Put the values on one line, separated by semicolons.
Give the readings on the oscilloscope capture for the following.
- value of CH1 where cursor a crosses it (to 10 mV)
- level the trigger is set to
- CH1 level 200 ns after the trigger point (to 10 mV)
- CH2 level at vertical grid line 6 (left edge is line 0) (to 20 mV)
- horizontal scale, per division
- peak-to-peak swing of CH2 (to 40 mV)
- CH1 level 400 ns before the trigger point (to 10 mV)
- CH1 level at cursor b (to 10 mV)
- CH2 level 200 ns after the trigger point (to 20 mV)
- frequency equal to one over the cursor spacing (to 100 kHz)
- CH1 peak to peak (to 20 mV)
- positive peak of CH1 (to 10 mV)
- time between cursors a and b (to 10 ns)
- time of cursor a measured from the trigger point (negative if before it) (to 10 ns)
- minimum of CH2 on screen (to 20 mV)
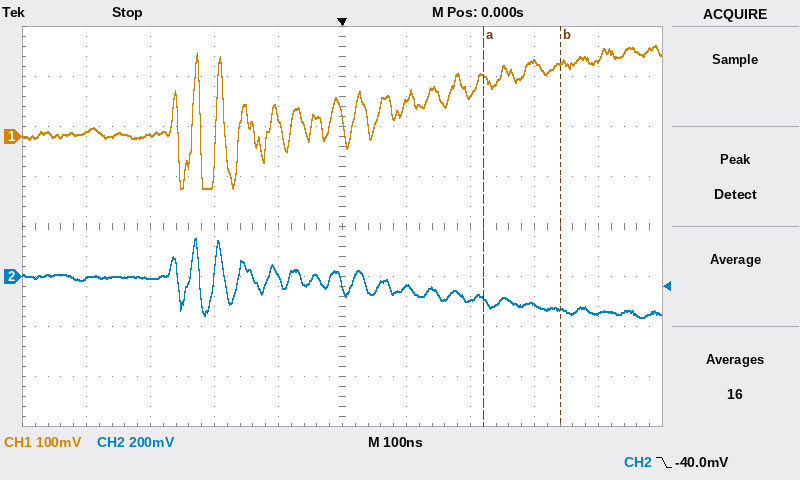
120 mV; -40.0 mV; 80 mV; -40 mV; 100 ns; 320 mV; 10 mV; 150 mV; -100 mV; 8.3 MHz; 280 mV; 180 mV; 120 ns; +220 ns; -160 mV
